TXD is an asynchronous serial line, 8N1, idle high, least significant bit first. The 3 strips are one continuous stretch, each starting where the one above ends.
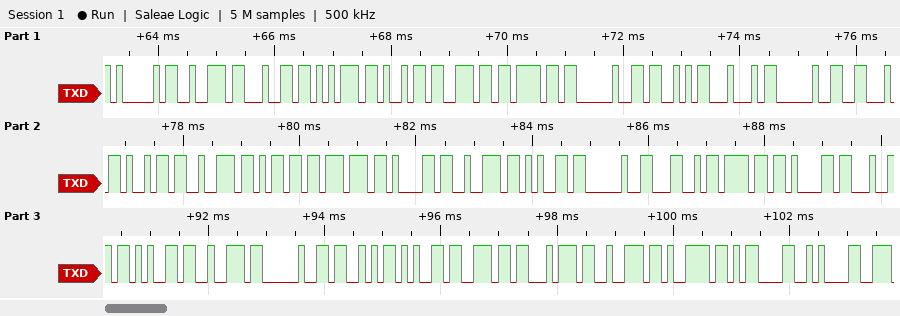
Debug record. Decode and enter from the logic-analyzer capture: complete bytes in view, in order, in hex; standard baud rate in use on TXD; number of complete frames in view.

41 72 64 75 69 6E 6F 20 53 44 20 46 69 72 6D 77 61 72 65 20 4C 6F 61 64 65 72 20 53 65 6E 74 72 79 0D 0A
9600 baud
35
